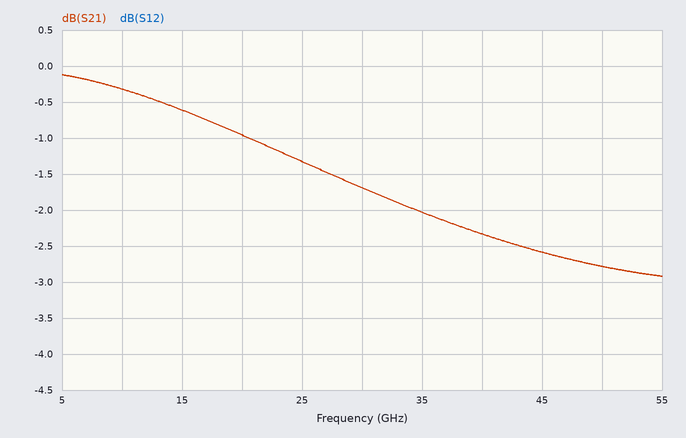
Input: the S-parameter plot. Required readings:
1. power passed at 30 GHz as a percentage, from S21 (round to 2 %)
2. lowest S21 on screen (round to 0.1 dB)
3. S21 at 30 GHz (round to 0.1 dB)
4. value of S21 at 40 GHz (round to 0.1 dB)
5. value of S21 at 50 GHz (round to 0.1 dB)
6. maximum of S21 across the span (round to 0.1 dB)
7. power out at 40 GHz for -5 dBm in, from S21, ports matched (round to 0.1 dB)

68 %
-2.9 dB
-1.7 dB
-2.3 dB
-2.8 dB
-0.1 dB
-7.3 dBm
